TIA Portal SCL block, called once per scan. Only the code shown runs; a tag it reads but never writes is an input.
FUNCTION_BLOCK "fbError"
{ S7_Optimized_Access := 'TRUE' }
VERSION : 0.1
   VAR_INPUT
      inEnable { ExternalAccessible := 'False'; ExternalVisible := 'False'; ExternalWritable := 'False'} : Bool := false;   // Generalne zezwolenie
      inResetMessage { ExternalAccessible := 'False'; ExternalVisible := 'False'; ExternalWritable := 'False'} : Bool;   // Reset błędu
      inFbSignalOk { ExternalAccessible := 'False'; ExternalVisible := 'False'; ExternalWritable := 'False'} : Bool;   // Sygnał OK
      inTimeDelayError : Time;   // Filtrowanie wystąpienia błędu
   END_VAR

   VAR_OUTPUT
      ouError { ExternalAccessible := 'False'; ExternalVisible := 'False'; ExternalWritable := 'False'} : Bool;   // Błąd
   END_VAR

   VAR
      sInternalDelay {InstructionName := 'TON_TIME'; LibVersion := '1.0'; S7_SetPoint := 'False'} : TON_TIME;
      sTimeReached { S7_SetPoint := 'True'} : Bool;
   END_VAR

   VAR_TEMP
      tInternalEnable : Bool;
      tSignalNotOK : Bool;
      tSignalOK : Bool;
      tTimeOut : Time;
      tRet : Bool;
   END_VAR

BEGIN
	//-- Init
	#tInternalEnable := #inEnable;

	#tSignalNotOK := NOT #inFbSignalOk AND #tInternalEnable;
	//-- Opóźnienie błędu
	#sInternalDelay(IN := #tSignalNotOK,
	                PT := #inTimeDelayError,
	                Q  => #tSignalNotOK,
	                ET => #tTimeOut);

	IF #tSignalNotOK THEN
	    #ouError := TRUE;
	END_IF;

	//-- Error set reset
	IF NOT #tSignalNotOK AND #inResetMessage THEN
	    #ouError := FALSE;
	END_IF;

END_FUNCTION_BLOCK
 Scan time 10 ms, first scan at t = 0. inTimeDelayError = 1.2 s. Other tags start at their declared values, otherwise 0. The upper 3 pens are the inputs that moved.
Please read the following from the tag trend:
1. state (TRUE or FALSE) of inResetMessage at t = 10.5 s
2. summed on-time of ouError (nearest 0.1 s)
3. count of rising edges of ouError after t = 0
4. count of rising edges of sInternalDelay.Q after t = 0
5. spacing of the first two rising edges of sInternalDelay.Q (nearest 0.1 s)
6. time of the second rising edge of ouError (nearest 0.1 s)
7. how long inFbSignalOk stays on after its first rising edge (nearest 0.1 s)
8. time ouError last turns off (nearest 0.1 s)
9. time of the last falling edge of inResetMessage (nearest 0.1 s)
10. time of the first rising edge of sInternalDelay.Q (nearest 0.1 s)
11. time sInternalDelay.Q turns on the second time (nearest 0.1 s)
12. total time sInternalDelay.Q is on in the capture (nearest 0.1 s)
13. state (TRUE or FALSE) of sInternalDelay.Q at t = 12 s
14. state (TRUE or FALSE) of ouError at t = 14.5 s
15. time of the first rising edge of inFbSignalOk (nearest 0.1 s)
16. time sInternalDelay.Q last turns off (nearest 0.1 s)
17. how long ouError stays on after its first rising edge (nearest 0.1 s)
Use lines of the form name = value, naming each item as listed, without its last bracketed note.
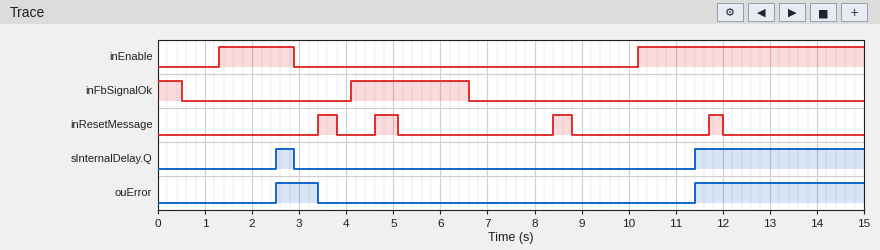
state (TRUE or FALSE) of inResetMessage at t = 10.5 s = FALSE
summed on-time of ouError = 4.5 s
count of rising edges of ouError after t = 0 = 2
count of rising edges of sInternalDelay.Q after t = 0 = 2
spacing of the first two rising edges of sInternalDelay.Q = 8.9 s
time of the second rising edge of ouError = 11.4 s
how long inFbSignalOk stays on after its first rising edge = 2.5 s
time ouError last turns off = 3.4 s
time of the last falling edge of inResetMessage = 12.0 s
time of the first rising edge of sInternalDelay.Q = 2.5 s
time sInternalDelay.Q turns on the second time = 11.4 s
total time sInternalDelay.Q is on in the capture = 4.0 s
state (TRUE or FALSE) of sInternalDelay.Q at t = 12 s = TRUE
state (TRUE or FALSE) of ouError at t = 14.5 s = TRUE
time of the first rising edge of inFbSignalOk = 4.1 s
time sInternalDelay.Q last turns off = 2.9 s
how long ouError stays on after its first rising edge = 0.9 s
